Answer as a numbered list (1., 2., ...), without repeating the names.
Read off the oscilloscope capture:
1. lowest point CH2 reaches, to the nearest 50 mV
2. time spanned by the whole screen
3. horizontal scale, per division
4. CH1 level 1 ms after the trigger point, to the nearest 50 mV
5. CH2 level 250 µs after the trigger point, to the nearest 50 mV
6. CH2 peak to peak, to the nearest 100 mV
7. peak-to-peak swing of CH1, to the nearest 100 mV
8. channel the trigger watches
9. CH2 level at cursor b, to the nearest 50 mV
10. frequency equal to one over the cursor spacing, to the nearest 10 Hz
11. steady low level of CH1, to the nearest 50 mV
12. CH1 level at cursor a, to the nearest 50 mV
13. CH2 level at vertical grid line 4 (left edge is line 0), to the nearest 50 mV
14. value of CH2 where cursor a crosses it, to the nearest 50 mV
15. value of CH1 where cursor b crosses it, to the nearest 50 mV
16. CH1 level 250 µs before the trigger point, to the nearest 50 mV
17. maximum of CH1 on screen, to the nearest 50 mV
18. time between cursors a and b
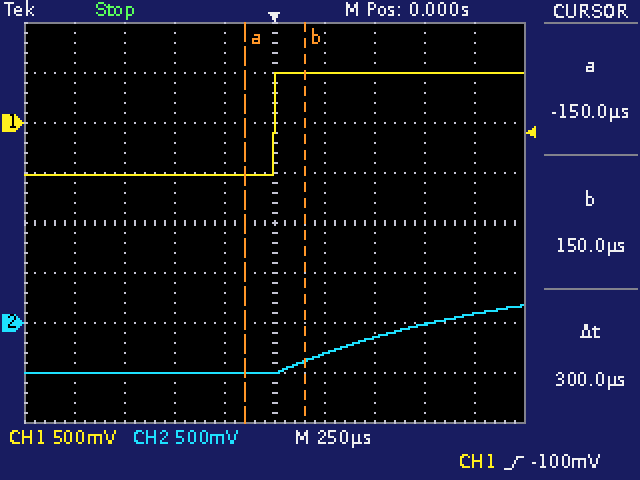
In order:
1. -500 mV
2. 2.5 ms
3. 250 µs
4. 500 mV
5. -300 mV
6. 700 mV
7. 1.00 V
8. CH1
9. -400 mV
10. 3.33 kHz
11. -500 mV
12. -500 mV
13. -500 mV
14. -500 mV
15. 500 mV
16. -500 mV
17. 500 mV
18. 300 µs
